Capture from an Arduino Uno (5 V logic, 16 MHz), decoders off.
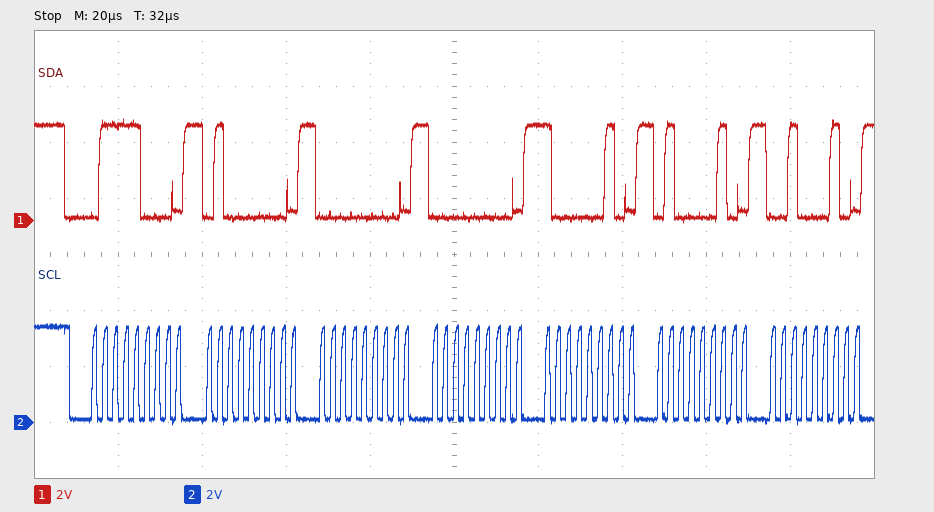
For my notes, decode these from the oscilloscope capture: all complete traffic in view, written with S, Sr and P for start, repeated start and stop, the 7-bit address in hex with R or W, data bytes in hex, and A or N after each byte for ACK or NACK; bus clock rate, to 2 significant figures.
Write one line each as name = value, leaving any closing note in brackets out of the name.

all complete traffic in view, written with S, Sr and P for start, repeated start and stop, the 7-bit address in hex with R or W, data bytes in hex, and A or N after each byte for ACK or NACK = S 3CW A 40 A 00 A 00 A 82 A 42 A 22 A
bus clock rate, to 2 significant figures = 400 kHz
